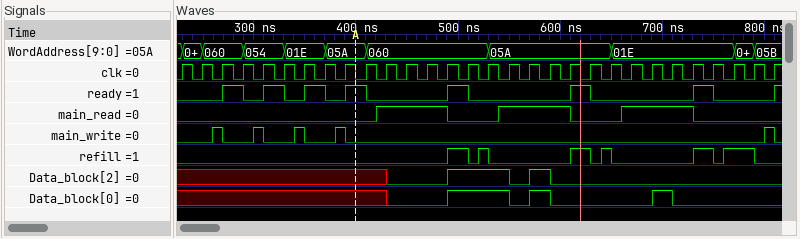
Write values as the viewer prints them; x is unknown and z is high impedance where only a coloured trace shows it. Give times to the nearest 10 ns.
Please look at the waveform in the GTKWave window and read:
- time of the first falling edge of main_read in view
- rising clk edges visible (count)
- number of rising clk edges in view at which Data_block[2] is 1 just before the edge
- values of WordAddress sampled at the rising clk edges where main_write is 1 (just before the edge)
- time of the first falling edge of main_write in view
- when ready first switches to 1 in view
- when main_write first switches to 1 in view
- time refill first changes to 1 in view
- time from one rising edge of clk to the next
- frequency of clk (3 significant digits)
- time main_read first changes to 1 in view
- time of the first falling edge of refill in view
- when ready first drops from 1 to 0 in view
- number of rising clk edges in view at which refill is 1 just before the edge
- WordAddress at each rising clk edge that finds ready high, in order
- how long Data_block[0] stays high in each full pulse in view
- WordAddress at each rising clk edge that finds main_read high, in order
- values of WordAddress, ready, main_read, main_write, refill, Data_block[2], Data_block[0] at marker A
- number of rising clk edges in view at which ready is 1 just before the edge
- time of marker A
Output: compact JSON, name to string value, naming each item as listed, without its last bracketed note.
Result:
{"time of the first falling edge of main_read in view": "490 ns", "rising clk edges visible": "30", "number of rising clk edges in view at which Data_block[2] is 1 just before the edge": "4", "values of WordAddress sampled at the rising clk edges where main_write is 1": "060, 054, 01E, 05A, 05B", "time of the first falling edge of main_write in view": "270 ns", "when ready first switches to 1 in view": "270 ns", "when main_write first switches to 1 in view": "260 ns", "time refill first changes to 1 in view": "490 ns", "time from one rising edge of clk to the next": "20 ns", "frequency of clk": "50.0 MHz", "time main_read first changes to 1 in view": "420 ns", "time of the first falling edge of refill in view": "510 ns", "when ready first drops from 1 to 0 in view": "290 ns", "number of rising clk edges in view at which refill is 1 just before the edge": "7", "WordAddress at each rising clk edge that finds ready high, in order": "060, 054, 01E, 05A, 060, 05A, 01E", "how long Data_block[0] stays high in each full pulse in view": "60 ns, 20 ns, 20 ns", "WordAddress at each rising clk edge that finds main_read high, in order": "060, 060, 060, 060, 05A, 05A, 05A, 05A, 01E, 01E, 01E, 01E", "values of WordAddress, ready, main_read, main_write, refill, Data_block[2], Data_block[0] at marker A": "WordAddress=05A, ready=1, main_read=0, main_write=0, refill=0, Data_block[2]=x, Data_block[0]=x", "number of rising clk edges in view at which ready is 1 just before the edge": "7", "time of marker A": "400 ns"}
